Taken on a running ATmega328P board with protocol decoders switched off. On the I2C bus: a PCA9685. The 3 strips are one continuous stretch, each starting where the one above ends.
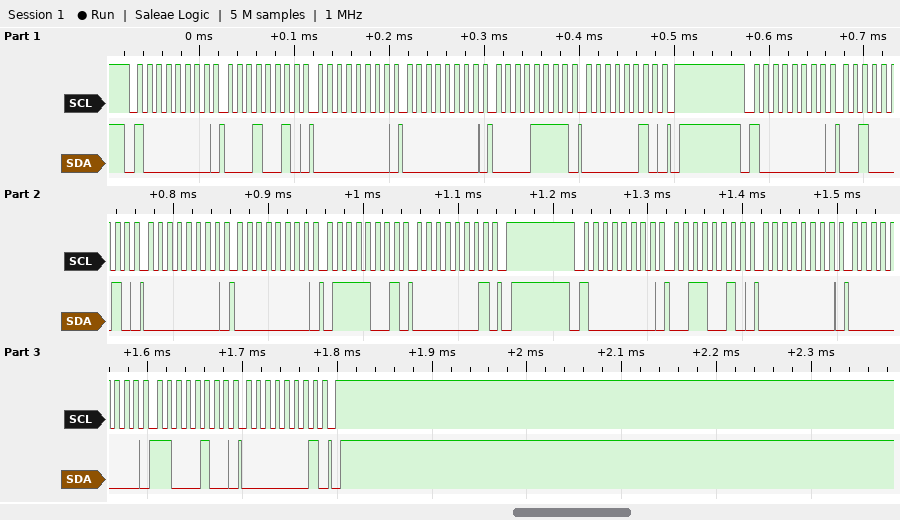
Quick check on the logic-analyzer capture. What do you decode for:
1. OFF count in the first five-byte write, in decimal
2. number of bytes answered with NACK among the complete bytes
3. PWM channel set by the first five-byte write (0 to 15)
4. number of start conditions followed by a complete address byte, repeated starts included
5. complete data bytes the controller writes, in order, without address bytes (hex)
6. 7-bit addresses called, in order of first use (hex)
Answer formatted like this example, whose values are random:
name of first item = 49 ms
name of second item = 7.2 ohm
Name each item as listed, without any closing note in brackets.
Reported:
OFF count in the first five-byte write, in decimal = 527
number of bytes answered with NACK among the complete bytes = 0
PWM channel set by the first five-byte write = 3
number of start conditions followed by a complete address byte, repeated starts included = 3
complete data bytes the controller writes, in order, without address bytes = 12 00 00 0F 02 22 00 00 79 01 32 00 00 C4 01
7-bit addresses called, in order of first use = 0x40
